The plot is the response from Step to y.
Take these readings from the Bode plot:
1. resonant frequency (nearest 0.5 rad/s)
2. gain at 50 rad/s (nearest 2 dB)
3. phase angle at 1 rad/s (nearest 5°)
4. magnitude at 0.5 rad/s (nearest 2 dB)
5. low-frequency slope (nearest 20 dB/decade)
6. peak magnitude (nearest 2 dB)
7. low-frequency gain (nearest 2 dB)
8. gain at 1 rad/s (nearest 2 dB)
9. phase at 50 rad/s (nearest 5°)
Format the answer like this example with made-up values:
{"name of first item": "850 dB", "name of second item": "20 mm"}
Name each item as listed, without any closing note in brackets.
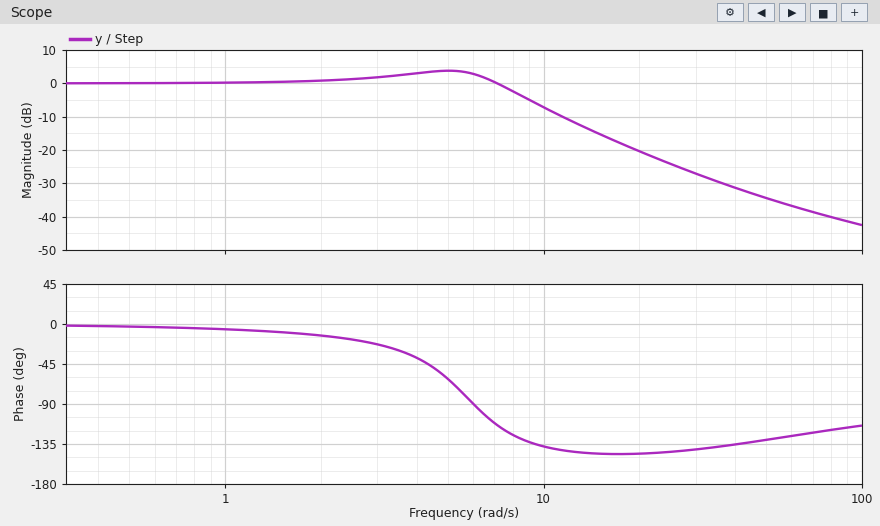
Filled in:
{"resonant frequency": "5.0 rad/s", "gain at 50 rad/s": "-34 dB", "phase angle at 1 rad/s": "-5°", "magnitude at 0.5 rad/s": "0 dB", "low-frequency slope": "0 dB/decade", "peak magnitude": "4 dB", "low-frequency gain": "0 dB", "gain at 1 rad/s": "0 dB", "phase at 50 rad/s": "-130°"}
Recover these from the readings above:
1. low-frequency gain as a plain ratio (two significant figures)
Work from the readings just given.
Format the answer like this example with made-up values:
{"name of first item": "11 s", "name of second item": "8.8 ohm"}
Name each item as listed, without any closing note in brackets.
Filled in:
{"low-frequency gain as a plain ratio": "1.0"}
